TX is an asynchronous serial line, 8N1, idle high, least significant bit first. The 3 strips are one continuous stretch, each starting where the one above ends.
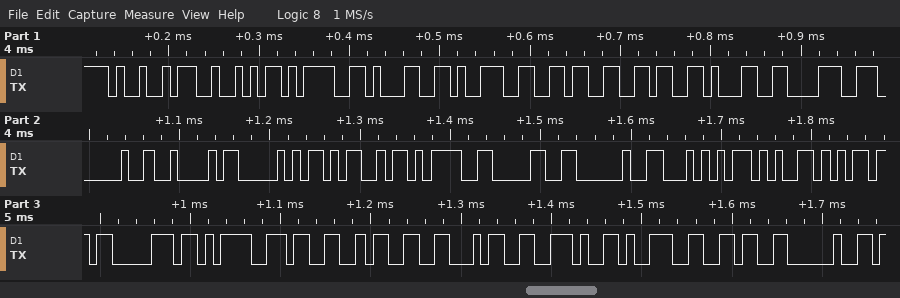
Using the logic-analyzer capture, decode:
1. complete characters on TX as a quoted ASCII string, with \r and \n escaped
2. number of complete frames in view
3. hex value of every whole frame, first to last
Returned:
"IR=196618 BPM=0 Temp=334.96 "
28
0x49 0x52 0x3D 0x31 0x39 0x36 0x36 0x31 0x38 0x20 0x42 0x50 0x4D 0x3D 0x30 0x20 0x54 0x65 0x6D 0x70 0x3D 0x33 0x33 0x34 0x2E 0x39 0x36 0x20
